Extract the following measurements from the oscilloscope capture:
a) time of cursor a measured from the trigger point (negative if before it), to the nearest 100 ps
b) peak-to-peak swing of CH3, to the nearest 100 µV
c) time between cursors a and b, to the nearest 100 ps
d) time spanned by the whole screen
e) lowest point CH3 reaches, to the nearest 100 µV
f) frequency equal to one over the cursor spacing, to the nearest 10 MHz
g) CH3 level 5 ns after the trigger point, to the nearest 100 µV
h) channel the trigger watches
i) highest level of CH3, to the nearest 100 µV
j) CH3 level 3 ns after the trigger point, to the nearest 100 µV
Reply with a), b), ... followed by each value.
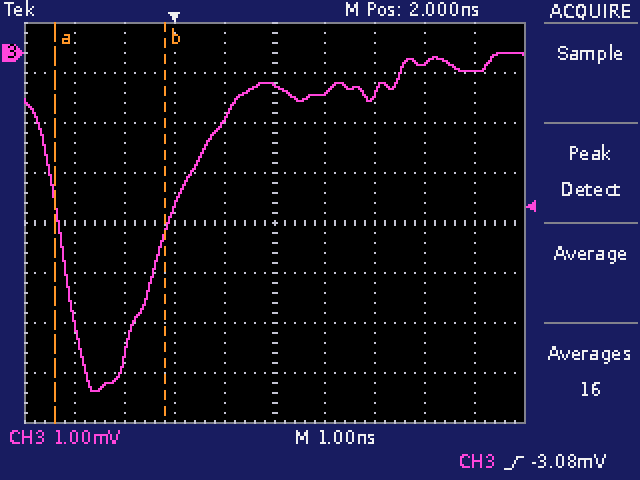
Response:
a) -2.4 ns
b) 6.8 mV
c) 2.2 ns
d) 10 ns
e) -6.8 mV
f) 450 MHz
g) -200 µV
h) CH3
i) 0.0 mV
j) -800 µV
